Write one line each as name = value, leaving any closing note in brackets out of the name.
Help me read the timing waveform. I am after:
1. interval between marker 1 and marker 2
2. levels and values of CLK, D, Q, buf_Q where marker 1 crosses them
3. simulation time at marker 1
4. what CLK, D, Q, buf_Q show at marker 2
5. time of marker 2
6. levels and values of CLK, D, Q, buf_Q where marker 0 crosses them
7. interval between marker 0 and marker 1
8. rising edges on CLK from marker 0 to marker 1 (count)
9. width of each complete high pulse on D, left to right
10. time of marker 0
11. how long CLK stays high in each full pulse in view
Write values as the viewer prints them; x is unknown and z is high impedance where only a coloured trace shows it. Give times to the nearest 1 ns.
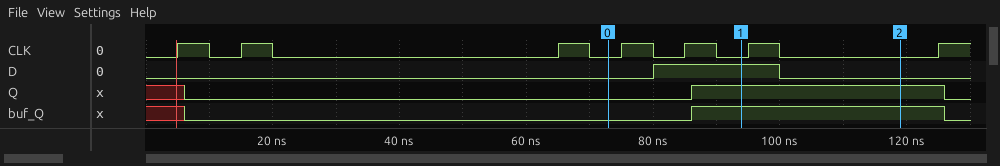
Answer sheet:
interval between marker 1 and marker 2 = 25 ns
levels and values of CLK, D, Q, buf_Q where marker 1 crosses them = CLK=0, D=1, Q=1, buf_Q=1
simulation time at marker 1 = 94 ns
what CLK, D, Q, buf_Q show at marker 2 = CLK=0, D=0, Q=1, buf_Q=1
time of marker 2 = 119 ns
levels and values of CLK, D, Q, buf_Q where marker 0 crosses them = CLK=0, D=0, Q=0, buf_Q=0
interval between marker 0 and marker 1 = 21 ns
rising edges on CLK from marker 0 to marker 1 = 2
width of each complete high pulse on D, left to right = 20 ns
time of marker 0 = 73 ns
how long CLK stays high in each full pulse in view = 5 ns, 5 ns, 5 ns, 5 ns, 5 ns, 5 ns
